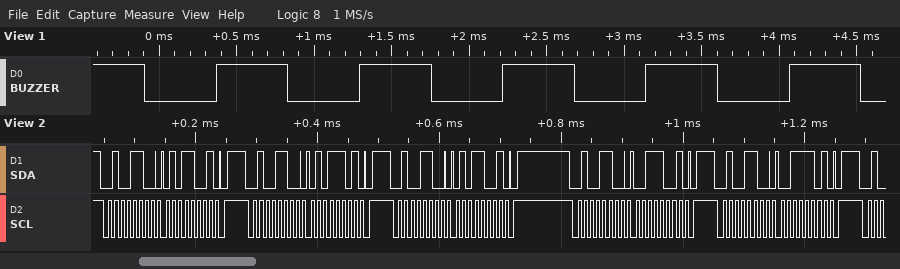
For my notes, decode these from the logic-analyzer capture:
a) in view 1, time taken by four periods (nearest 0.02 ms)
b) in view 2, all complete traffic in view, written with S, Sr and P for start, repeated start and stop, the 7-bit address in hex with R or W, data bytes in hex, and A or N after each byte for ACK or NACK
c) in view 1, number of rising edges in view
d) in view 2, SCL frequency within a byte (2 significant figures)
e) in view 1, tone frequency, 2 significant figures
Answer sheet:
3.70 ms
S 26W A 59 A P S 26W A 5D A P S 26W A 59 A P S 26W A 39 A P S 26W A 3D A P
5
100 kHz
1.1 kHz
